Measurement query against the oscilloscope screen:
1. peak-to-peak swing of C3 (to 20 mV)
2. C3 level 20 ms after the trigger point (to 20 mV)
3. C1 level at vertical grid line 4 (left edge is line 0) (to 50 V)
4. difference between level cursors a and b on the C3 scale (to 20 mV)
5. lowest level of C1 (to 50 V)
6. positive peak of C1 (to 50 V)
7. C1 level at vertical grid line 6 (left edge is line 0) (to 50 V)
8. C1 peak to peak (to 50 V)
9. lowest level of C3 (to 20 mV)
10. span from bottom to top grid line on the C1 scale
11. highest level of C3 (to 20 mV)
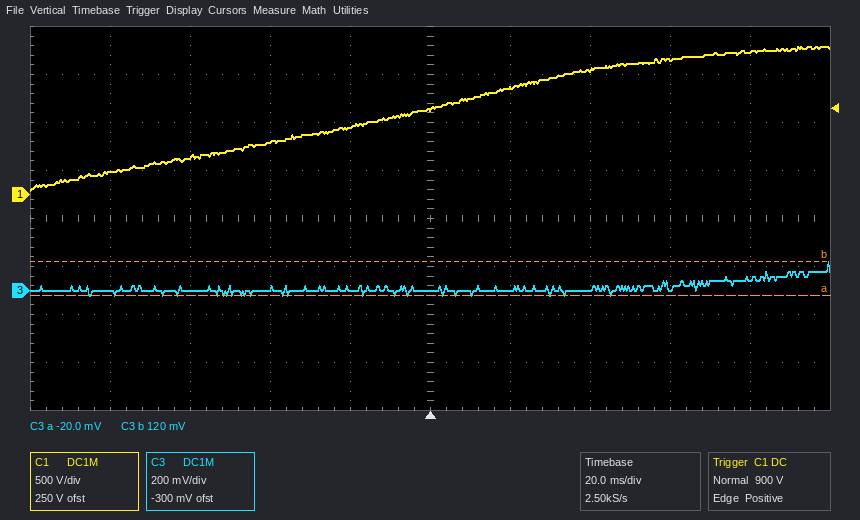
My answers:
140 mV
0 mV
700 V
140 mV
50 V
1.55 kV
1.10 kV
1.50 kV
-20 mV
4 kV
120 mV
